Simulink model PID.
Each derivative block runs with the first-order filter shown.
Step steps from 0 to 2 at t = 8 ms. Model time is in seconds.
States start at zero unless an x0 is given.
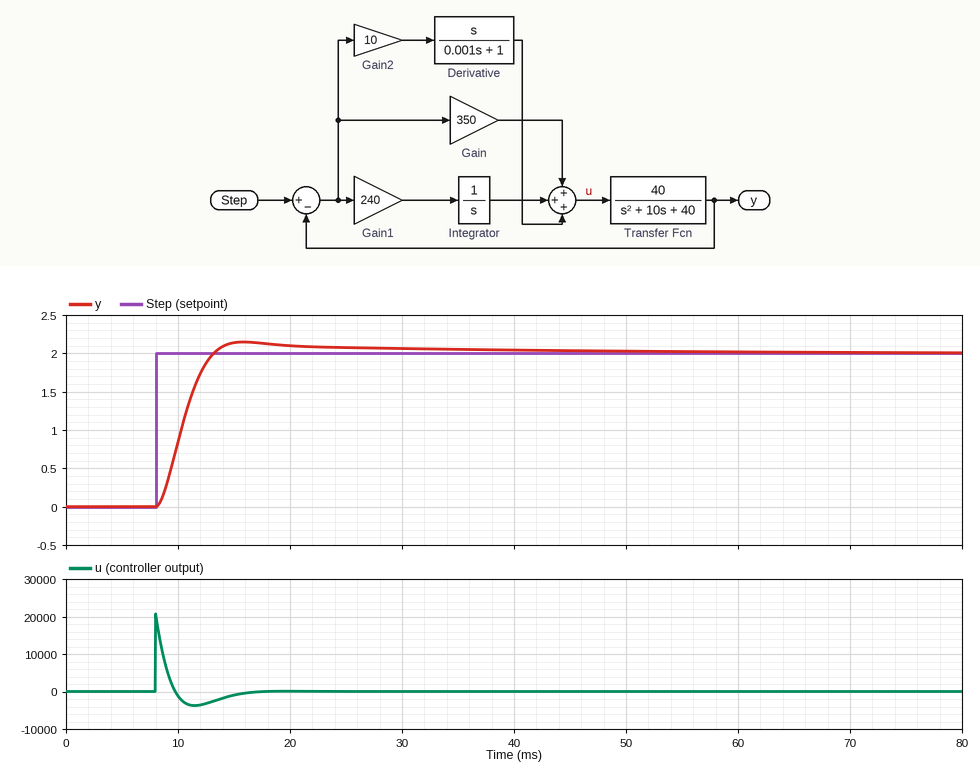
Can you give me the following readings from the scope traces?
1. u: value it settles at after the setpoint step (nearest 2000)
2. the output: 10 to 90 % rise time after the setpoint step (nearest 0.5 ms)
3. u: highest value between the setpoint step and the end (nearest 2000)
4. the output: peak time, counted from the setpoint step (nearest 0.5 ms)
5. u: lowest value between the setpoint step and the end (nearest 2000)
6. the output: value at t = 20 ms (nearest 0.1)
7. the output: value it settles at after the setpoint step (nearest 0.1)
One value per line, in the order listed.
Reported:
0
3.5 ms
20000
8.0 ms
-4000
2.1
2.0
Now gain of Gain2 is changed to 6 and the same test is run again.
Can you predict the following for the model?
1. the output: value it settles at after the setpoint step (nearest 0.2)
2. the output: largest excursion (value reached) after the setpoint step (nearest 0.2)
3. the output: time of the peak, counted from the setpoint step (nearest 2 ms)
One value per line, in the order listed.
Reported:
2.0
2.2
14 ms
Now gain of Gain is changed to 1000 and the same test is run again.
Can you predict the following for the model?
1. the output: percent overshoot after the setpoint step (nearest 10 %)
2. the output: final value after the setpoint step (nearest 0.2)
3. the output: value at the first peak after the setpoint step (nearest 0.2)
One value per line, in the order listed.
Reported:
20 %
2.0
2.4
